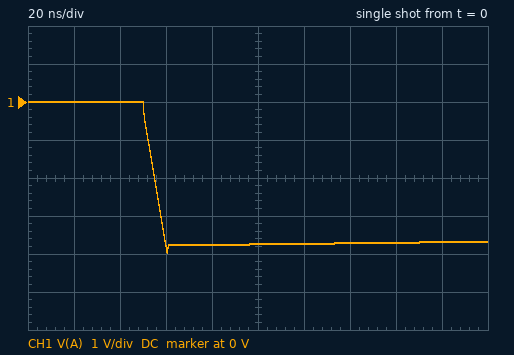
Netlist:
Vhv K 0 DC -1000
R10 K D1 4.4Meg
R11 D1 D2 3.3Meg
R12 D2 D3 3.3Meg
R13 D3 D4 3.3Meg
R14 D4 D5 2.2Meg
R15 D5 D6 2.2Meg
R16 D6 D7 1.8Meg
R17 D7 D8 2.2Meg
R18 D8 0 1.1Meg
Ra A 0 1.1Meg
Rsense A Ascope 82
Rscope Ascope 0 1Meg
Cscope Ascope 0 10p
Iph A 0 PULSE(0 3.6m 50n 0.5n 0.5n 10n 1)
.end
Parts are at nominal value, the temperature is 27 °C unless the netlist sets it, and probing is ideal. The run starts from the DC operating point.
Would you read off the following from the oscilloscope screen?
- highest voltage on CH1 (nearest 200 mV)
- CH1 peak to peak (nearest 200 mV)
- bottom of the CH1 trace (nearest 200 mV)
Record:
0 V
4.0 V
-4.0 V
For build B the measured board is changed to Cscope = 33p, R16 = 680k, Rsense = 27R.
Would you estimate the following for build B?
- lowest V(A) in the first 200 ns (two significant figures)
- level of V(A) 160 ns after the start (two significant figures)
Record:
-1.2 V
-1.1 V
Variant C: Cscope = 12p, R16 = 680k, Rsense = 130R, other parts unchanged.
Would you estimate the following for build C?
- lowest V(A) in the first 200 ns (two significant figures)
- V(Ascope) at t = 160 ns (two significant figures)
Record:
-3.5 V
-3.1 V
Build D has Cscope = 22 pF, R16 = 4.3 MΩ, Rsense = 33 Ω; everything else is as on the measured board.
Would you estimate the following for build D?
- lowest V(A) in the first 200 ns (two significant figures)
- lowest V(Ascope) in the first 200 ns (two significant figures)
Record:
-1.8 V
-1.7 V
